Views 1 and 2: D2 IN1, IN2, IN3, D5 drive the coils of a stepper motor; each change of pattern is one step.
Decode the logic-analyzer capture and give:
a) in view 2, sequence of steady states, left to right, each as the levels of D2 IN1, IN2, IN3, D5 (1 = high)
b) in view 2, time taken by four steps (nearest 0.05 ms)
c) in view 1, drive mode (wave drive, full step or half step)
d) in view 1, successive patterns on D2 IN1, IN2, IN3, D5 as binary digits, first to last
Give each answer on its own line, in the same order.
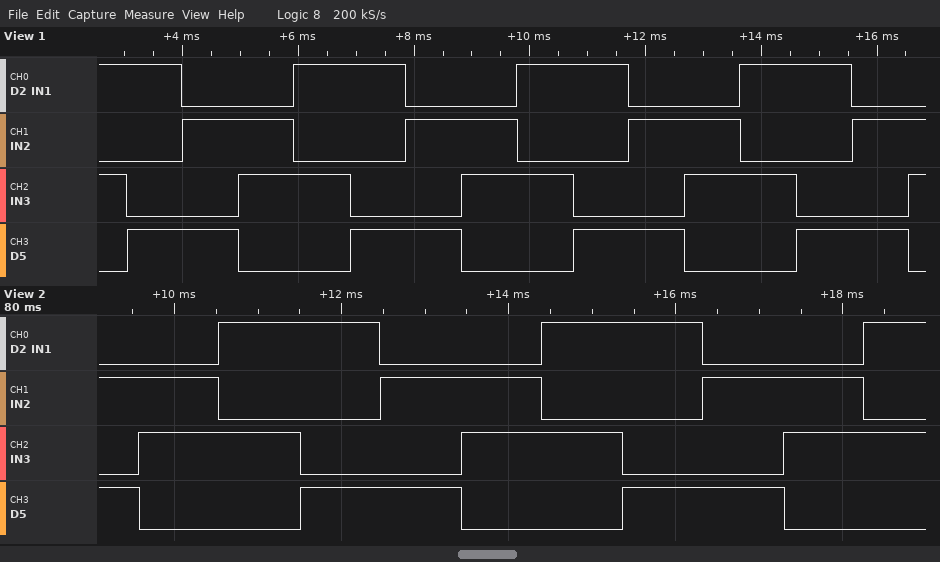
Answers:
0101 0110 1010 1001 0101 0110 1010 1001 0101 0110 1010
3.85 ms
full step
1010 1001 0101 0110 1010 1001 0101 0110 1010 1001 0101 0110 1010 1001 0101 0110
